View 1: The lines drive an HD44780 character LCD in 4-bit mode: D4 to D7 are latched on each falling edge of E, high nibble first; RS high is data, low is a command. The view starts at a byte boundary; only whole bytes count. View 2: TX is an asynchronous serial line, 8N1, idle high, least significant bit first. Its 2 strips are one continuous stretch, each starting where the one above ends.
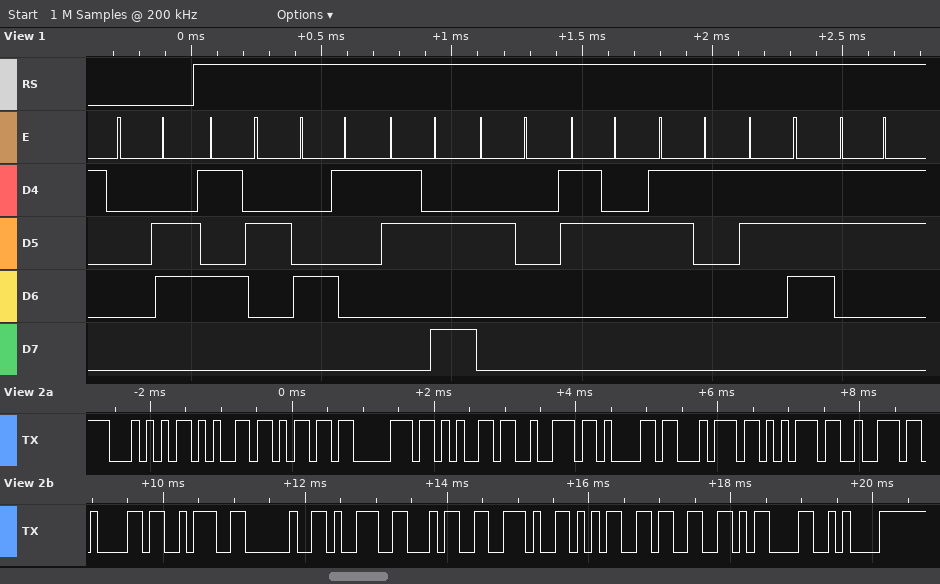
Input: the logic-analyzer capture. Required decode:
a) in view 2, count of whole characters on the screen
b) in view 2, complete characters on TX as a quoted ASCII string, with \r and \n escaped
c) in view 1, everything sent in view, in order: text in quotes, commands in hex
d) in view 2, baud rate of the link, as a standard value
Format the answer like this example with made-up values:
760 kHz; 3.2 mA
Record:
20; "Temperatura: 94.53\r\n"; 0x06 "RA: 2173"; 9600 baud
